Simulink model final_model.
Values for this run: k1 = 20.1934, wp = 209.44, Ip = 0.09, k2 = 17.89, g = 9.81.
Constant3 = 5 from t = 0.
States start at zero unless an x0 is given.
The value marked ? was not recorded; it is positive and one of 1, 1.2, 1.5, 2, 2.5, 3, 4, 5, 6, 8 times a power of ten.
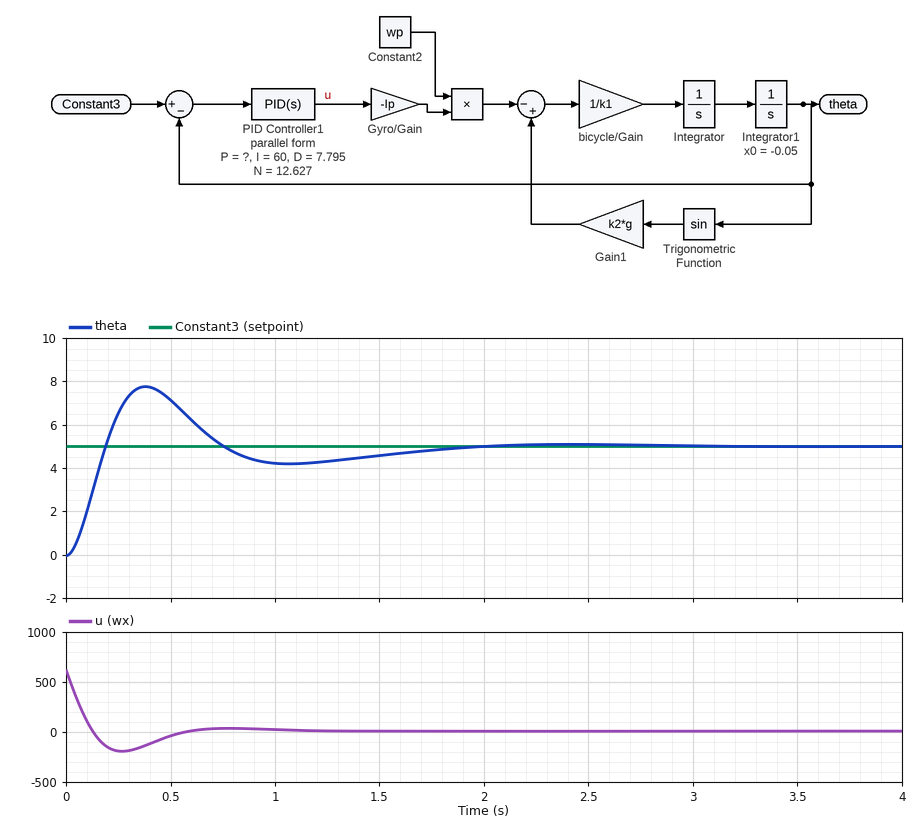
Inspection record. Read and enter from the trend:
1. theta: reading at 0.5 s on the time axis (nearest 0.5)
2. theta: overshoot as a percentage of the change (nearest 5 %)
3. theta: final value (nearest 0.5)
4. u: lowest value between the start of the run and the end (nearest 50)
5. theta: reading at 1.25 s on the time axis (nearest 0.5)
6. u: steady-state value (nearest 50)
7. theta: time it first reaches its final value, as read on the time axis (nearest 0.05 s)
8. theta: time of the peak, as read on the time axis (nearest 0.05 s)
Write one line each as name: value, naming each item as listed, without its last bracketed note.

theta: reading at 0.5 s on the time axis: 7.0
theta: overshoot as a percentage of the change: 55 %
theta: final value: 5.0
u: lowest value between the start of the run and the end: -200
theta: reading at 1.25 s on the time axis: 4.5
u: steady-state value: 0
theta: time it first reaches its final value, as read on the time axis: 0.20 s
theta: time of the peak, as read on the time axis: 0.40 s
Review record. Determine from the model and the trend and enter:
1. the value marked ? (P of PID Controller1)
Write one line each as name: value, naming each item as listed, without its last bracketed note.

the value marked ?: 25
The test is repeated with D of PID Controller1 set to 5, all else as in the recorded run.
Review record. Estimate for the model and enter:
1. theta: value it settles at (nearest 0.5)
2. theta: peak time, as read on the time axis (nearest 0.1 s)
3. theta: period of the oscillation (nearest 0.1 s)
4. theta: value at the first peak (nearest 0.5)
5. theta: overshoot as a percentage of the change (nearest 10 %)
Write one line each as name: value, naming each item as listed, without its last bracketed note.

theta: value it settles at: 5.0
theta: peak time, as read on the time axis: 0.5 s
theta: period of the oscillation: 1.2 s
theta: value at the first peak: 8.5
theta: overshoot as a percentage of the change: 70 %
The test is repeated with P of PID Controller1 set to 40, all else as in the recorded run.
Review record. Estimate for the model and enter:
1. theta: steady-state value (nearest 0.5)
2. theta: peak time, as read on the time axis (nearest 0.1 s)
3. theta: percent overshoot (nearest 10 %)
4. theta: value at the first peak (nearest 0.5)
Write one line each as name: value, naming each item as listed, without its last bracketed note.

theta: steady-state value: 5.0
theta: peak time, as read on the time axis: 0.3 s
theta: percent overshoot: 60 %
theta: value at the first peak: 8.0
